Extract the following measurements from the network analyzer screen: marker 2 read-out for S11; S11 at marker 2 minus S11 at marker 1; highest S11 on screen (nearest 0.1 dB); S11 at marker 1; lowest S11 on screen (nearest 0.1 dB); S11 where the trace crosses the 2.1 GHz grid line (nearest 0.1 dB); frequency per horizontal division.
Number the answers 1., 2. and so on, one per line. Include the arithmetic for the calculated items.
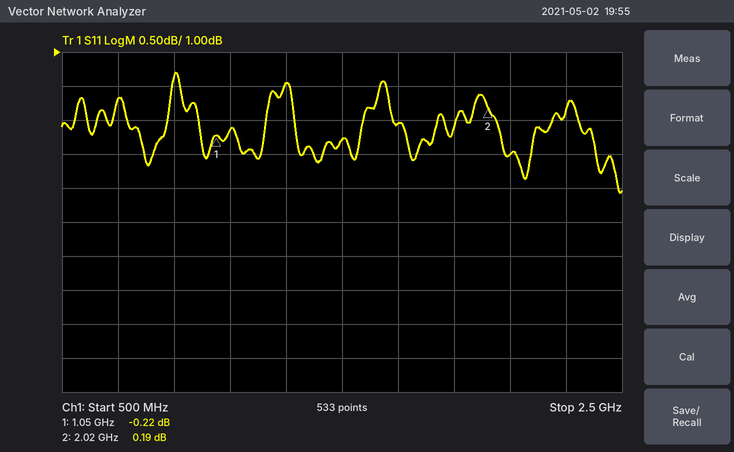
1. 0.19 dB
2. 0.19 − (-0.22) = 0.41 dB
3. 0.7 dB
4. -0.22 dB
5. -1.1 dB
6. -0.5 dB
7. 200 MHz
